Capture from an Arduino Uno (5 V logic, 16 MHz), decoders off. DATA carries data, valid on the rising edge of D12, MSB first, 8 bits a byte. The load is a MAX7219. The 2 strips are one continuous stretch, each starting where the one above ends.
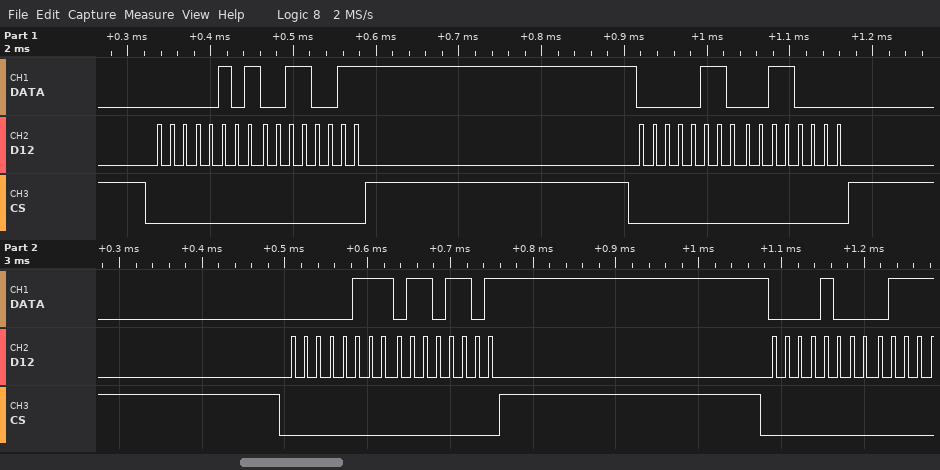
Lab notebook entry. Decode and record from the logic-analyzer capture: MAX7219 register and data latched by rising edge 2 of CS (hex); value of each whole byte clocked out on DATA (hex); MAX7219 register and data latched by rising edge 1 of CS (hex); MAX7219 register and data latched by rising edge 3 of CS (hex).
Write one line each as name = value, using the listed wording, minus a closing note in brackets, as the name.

MAX7219 register and data latched by rising edge 2 of CS = register 0x6, data 0x30
value of each whole byte clocked out on DATA = 05 33 06 30 07 6D 08
MAX7219 register and data latched by rising edge 1 of CS = register 0x5, data 0x33
MAX7219 register and data latched by rising edge 3 of CS = register 0x7, data 0x6D
